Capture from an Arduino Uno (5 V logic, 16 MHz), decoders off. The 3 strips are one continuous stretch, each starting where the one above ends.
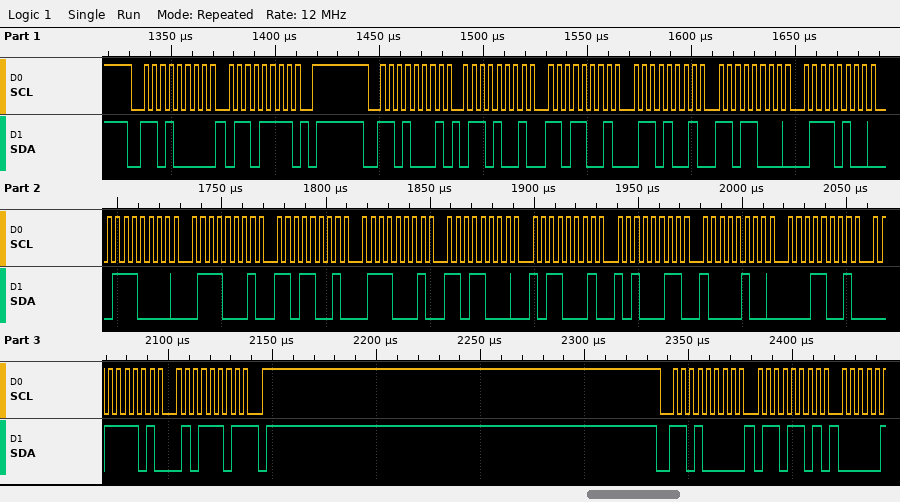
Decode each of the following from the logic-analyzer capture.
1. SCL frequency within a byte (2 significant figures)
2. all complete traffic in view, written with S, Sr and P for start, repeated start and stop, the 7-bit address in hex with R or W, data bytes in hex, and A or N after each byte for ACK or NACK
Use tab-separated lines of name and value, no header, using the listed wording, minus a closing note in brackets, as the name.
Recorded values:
SCL frequency within a byte	250 kHz
all complete traffic in view, written with S, Sr and P for start, repeated start and stop, the 7-bit address in hex with R or W, data bytes in hex, and A or N after each byte for ACK or NACK	S 68W A 6F A P S 68R A 69 A D9 A 69 A D8 A 74 A 70 A 71 A D9 A 71 A D8 A B1 A A3 A 84 A 19 A 3D A 5D N P S 68W A 6D A
